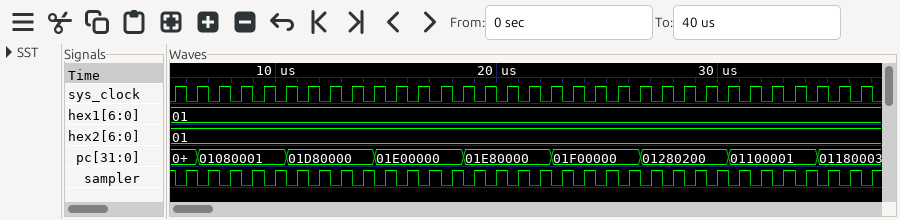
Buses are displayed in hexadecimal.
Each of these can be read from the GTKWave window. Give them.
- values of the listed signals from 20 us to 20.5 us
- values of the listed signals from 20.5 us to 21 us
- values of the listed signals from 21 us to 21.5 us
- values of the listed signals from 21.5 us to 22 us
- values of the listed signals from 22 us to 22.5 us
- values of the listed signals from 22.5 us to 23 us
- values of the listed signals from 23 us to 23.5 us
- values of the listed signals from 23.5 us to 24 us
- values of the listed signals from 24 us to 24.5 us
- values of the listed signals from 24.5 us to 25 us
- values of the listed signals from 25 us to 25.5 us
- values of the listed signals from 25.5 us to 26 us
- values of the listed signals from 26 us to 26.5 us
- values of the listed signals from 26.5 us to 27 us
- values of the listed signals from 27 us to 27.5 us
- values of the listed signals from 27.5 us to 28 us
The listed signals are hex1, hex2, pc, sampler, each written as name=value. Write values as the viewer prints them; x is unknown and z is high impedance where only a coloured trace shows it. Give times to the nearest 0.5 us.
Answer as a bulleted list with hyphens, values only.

- hex1=01, hex2=01, pc=01E80000, sampler=1
- hex1=01, hex2=01, pc=01E80000, sampler=0
- hex1=01, hex2=01, pc=01E80000, sampler=1
- hex1=01, hex2=01, pc=01E80000, sampler=0
- hex1=01, hex2=01, pc=01E80000, sampler=1
- hex1=01, hex2=01, pc=01F00000, sampler=0
- hex1=01, hex2=01, pc=01F00000, sampler=1
- hex1=01, hex2=01, pc=01F00000, sampler=0
- hex1=01, hex2=01, pc=01F00000, sampler=1
- hex1=01, hex2=01, pc=01F00000, sampler=0
- hex1=01, hex2=01, pc=01F00000, sampler=1
- hex1=01, hex2=01, pc=01F00000, sampler=0
- hex1=01, hex2=01, pc=01F00000, sampler=1
- hex1=01, hex2=01, pc=01280200, sampler=0
- hex1=01, hex2=01, pc=01280200, sampler=1
- hex1=01, hex2=01, pc=01280200, sampler=0
